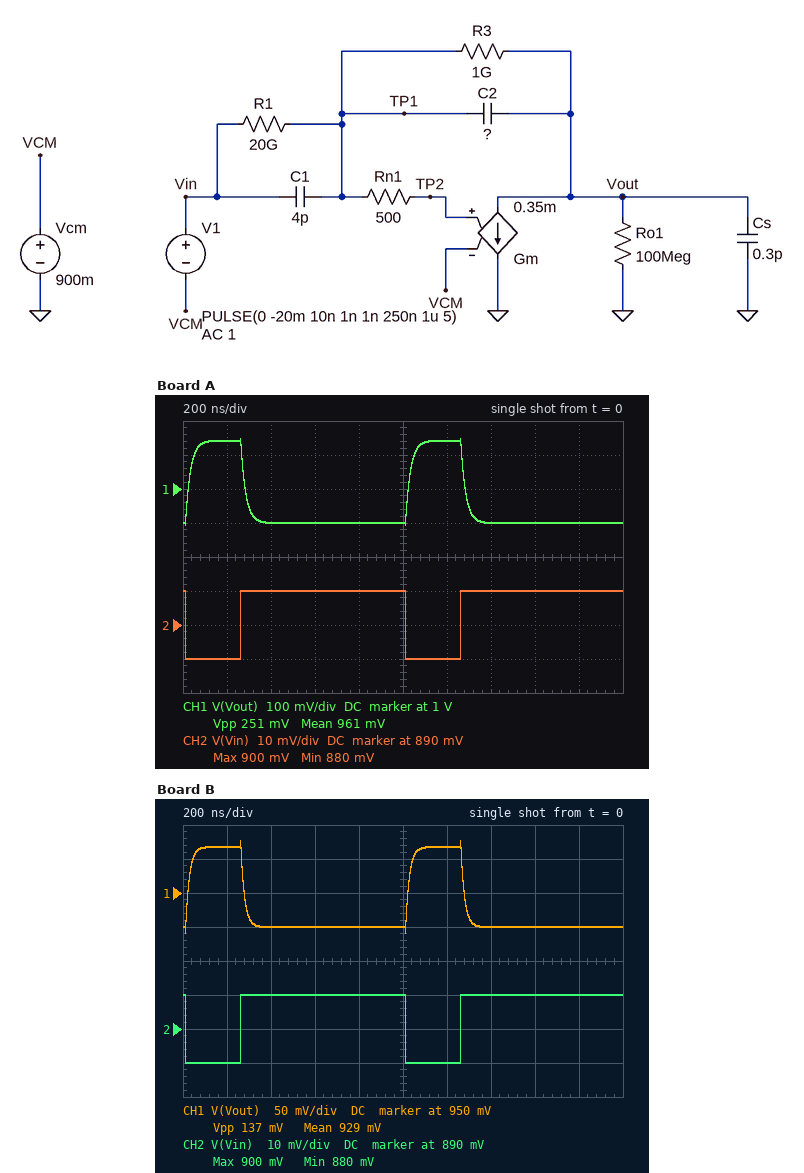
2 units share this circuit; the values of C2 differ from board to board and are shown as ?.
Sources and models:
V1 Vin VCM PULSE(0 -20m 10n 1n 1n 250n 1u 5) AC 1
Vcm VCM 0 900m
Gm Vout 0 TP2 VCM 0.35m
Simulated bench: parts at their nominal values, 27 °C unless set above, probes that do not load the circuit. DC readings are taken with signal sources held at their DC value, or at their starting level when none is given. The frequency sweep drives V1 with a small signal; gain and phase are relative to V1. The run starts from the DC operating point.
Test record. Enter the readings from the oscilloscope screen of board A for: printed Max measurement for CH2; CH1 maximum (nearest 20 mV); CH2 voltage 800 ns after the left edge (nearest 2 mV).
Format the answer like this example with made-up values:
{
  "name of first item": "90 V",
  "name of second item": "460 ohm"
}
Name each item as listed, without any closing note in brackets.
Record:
{
  "printed Max measurement for CH2": "900 mV",
  "CH1 maximum": "1.14 V",
  "CH2 voltage 800 ns after the left edge": "900 mV"
}
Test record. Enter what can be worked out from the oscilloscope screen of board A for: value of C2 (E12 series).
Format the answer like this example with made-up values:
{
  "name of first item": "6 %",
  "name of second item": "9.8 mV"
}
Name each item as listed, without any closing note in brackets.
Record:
{
  "value of C2": "330 fF"
}
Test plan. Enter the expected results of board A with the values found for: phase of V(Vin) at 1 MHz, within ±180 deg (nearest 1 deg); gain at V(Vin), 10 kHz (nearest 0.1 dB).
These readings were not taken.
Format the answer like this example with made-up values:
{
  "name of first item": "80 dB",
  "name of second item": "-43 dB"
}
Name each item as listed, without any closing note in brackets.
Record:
{
  "phase of V(Vin) at 1 MHz, within ±180 deg": "0 deg",
  "gain at V(Vin), 10 kHz": "0 dB"
}
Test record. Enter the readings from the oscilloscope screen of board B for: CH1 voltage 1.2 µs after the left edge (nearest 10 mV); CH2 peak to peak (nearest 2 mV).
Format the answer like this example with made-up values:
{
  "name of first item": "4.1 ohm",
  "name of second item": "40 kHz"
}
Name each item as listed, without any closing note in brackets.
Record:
{
  "CH1 voltage 1.2 µs after the left edge": "1.02 V",
  "CH2 peak to peak": "20 mV"
}
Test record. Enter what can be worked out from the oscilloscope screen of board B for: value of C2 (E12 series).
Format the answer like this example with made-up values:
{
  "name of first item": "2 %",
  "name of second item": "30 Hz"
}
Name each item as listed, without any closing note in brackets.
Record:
{
  "value of C2": "680 fF"
}
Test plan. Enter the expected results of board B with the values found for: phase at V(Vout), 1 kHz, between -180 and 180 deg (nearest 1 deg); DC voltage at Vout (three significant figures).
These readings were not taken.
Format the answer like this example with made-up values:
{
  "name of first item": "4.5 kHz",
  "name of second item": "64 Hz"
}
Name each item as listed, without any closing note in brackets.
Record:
{
  "phase at V(Vout), 1 kHz, between -180 and 180 deg": "-167 deg",
  "DC voltage at Vout": "900 mV"
}
